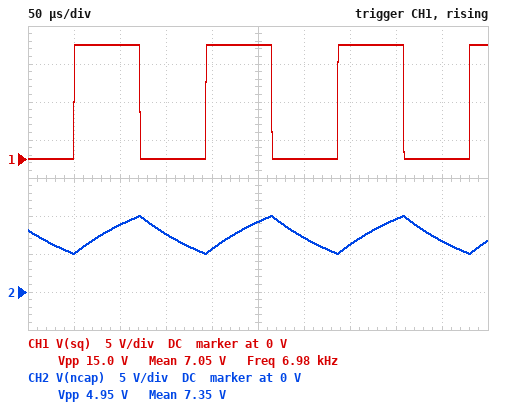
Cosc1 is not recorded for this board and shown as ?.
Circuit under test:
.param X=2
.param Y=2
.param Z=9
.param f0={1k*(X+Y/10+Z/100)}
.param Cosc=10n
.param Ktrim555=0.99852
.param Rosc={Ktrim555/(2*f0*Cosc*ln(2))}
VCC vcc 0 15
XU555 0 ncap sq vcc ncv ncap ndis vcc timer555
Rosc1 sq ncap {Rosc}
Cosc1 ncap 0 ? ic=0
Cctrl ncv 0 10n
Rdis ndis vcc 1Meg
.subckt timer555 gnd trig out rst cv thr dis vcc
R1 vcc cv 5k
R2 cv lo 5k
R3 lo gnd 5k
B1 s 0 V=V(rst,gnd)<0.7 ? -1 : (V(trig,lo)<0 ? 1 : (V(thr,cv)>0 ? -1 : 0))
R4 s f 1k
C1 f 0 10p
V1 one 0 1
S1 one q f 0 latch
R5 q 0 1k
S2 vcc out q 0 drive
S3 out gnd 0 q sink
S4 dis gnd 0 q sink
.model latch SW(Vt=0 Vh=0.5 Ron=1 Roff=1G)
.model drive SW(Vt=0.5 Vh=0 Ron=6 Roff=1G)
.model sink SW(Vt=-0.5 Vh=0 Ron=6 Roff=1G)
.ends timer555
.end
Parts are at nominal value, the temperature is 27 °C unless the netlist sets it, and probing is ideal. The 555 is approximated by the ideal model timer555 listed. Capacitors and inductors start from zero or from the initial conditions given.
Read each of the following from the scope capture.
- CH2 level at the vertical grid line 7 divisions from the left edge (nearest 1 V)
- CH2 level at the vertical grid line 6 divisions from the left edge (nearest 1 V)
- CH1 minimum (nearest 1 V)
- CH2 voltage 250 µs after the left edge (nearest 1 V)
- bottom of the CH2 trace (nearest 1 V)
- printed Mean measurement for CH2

6 V
7 V
0 V
9 V
5 V
7.35 V
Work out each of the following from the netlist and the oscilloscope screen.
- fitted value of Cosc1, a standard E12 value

3.3 nF
